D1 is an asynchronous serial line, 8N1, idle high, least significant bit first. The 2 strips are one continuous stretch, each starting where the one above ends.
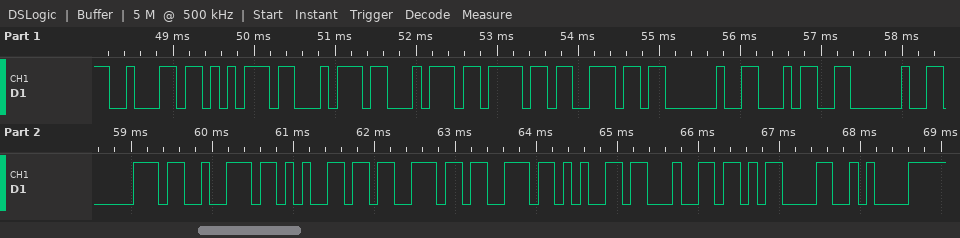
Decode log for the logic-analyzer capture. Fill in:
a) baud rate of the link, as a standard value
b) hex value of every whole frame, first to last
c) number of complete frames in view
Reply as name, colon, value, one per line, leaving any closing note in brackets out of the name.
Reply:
baud rate of the link, as a standard value: 9600 baud
hex value of every whole frame, first to last: 62 75 74 74 6F 6E 20 34 20 70 72 65 73 73 65 64 0D 0A
number of complete frames in view: 18
